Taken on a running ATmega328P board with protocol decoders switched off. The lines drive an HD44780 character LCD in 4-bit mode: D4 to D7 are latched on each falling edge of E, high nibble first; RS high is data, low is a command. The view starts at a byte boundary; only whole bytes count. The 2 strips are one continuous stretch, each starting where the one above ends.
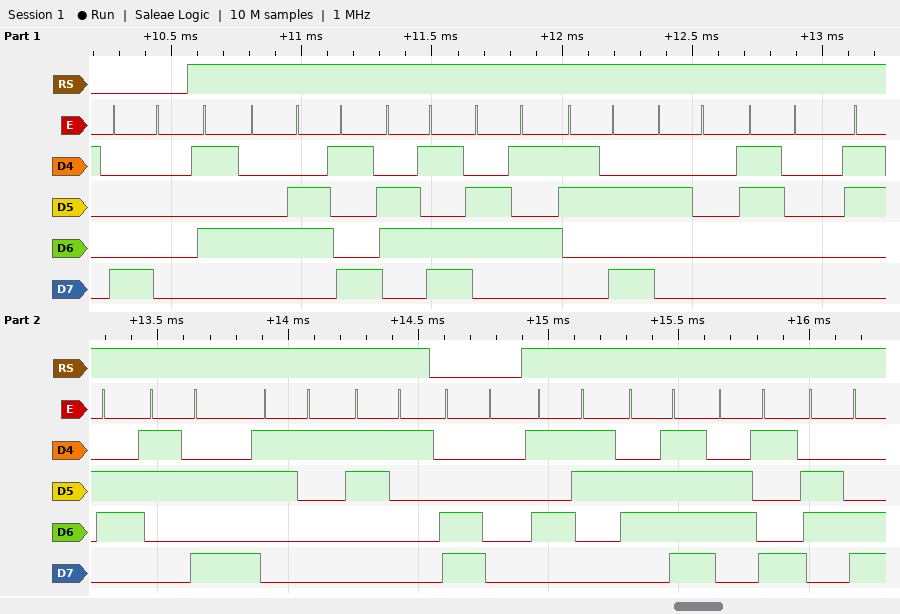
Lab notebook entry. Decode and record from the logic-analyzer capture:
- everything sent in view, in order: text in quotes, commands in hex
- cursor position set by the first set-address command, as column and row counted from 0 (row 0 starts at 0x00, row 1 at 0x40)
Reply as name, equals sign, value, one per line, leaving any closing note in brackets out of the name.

everything sent in view, in order: text in quotes, commands in hex = 0x80 "Time: 06:11" 0xC0 "Soil"
cursor position set by the first set-address command, as column and row counted from 0 = column 0, row 0
